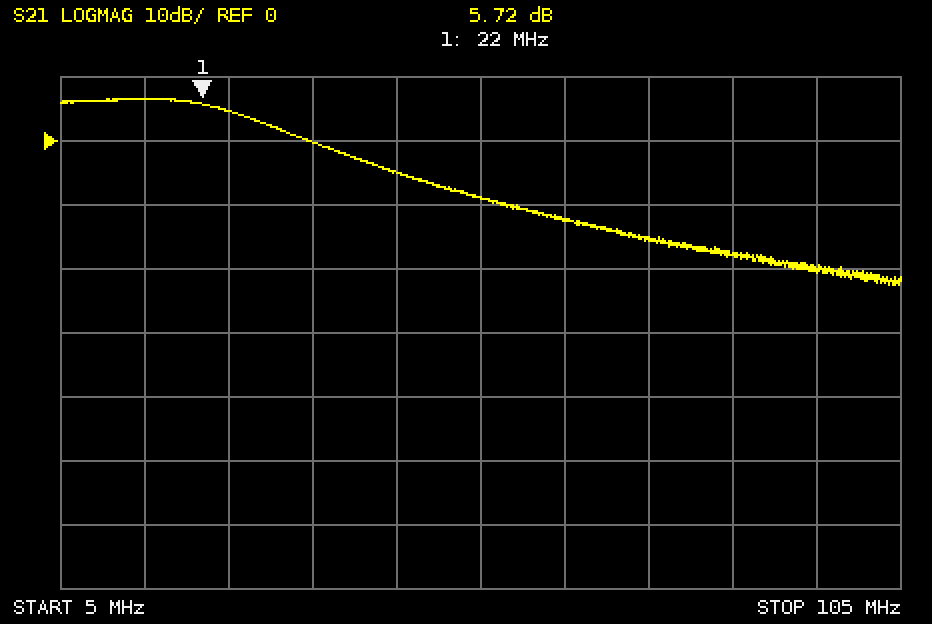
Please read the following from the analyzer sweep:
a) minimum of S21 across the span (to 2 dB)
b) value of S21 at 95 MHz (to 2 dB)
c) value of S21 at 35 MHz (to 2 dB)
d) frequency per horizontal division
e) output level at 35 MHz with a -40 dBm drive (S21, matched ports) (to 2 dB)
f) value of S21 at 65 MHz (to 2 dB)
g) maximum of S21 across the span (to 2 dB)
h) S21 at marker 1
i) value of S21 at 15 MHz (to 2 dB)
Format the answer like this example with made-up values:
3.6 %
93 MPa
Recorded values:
-22 dB
-20 dB
0 dB
10 MHz
-40 dBm
-12 dB
6 dB
5.72 dB
6 dB
